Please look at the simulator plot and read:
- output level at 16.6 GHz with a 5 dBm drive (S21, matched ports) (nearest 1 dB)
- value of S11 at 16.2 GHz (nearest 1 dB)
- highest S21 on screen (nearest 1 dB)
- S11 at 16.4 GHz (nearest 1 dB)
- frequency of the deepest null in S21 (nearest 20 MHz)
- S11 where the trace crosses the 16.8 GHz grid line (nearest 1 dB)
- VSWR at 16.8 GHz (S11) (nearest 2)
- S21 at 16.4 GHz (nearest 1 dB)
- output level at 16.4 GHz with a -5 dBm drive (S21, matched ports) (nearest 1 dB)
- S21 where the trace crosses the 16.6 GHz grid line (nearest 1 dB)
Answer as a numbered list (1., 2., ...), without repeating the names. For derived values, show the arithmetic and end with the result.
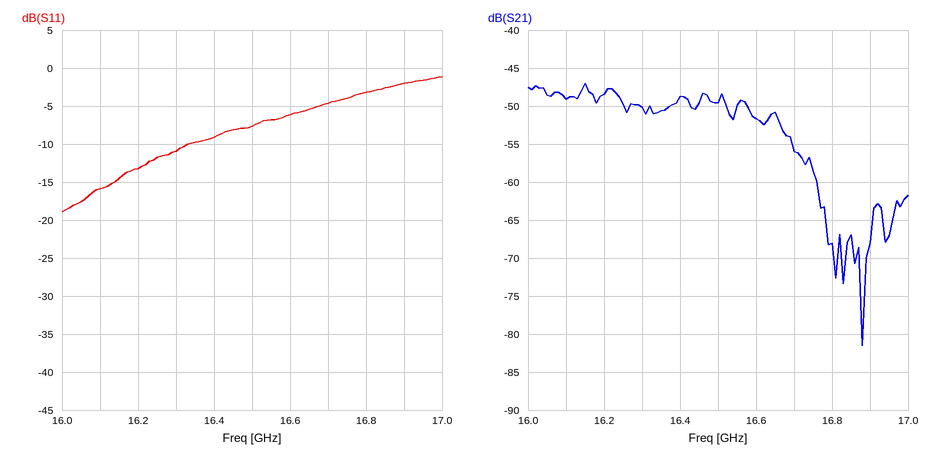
1. 5 dBm + (-52 dB) = -47 dBm
2. -13 dB
3. -47 dB
4. -9 dB
5. 16.88 GHz
6. -3 dB
7. |Γ| = 10^(-3/20) = 0.7079; VSWR = (1 + 0.7079)/(1 − 0.7079) ≈ 6
8. -49 dB
9. -5 dBm + (-49 dB) = -54 dBm
10. -52 dB
